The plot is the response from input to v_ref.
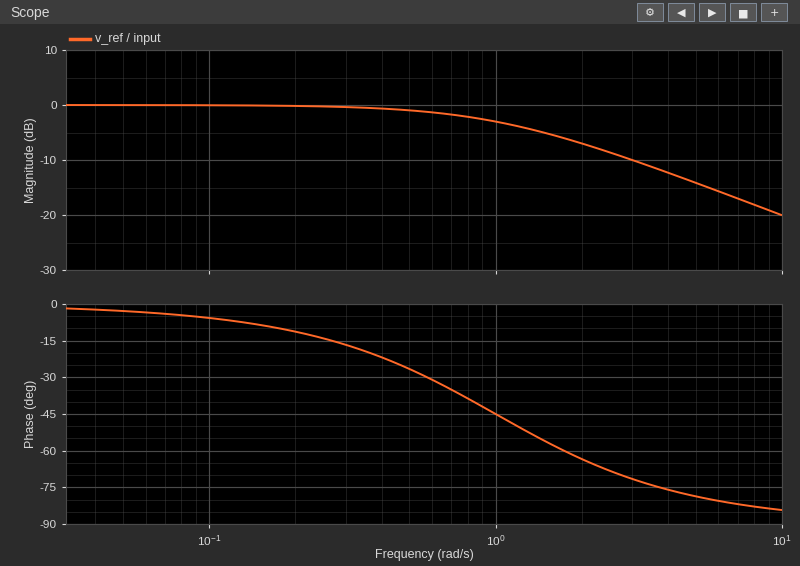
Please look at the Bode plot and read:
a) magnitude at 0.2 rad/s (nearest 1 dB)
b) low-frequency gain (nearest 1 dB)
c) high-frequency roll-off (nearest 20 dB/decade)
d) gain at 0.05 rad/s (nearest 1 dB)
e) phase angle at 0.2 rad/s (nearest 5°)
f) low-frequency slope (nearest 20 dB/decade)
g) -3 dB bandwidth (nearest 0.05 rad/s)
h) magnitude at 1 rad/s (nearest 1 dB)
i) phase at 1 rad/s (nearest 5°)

0 dB
0 dB
-20 dB/decade
0 dB
-10°
0 dB/decade
1.00 rad/s
-3 dB
-45°
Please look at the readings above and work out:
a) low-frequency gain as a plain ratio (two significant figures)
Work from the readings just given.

1.0
